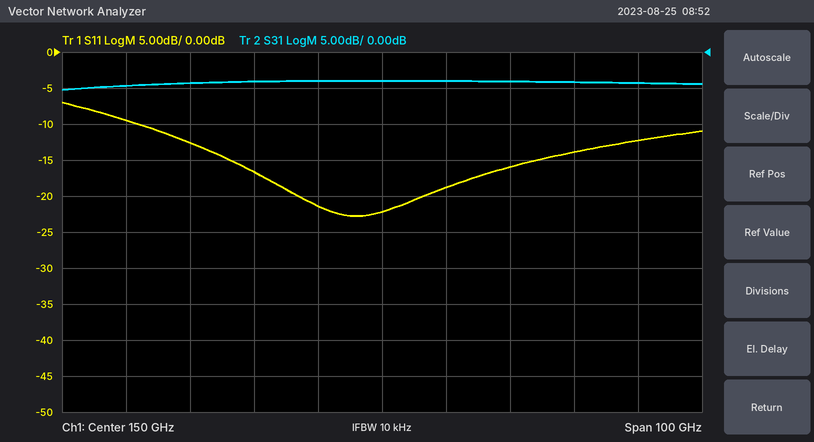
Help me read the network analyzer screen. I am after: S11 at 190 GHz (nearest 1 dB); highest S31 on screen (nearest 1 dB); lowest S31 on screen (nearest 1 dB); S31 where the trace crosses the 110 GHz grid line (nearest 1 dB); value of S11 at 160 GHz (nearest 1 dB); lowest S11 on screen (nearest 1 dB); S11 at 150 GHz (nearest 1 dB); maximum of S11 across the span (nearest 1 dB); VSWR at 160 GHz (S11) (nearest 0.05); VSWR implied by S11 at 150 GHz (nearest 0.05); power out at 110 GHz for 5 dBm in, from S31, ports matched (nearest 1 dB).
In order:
-12 dB
-4 dB
-5 dB
-5 dB
-19 dB
-23 dB
-22 dB
-7 dB
1.25
1.15
0 dBm
